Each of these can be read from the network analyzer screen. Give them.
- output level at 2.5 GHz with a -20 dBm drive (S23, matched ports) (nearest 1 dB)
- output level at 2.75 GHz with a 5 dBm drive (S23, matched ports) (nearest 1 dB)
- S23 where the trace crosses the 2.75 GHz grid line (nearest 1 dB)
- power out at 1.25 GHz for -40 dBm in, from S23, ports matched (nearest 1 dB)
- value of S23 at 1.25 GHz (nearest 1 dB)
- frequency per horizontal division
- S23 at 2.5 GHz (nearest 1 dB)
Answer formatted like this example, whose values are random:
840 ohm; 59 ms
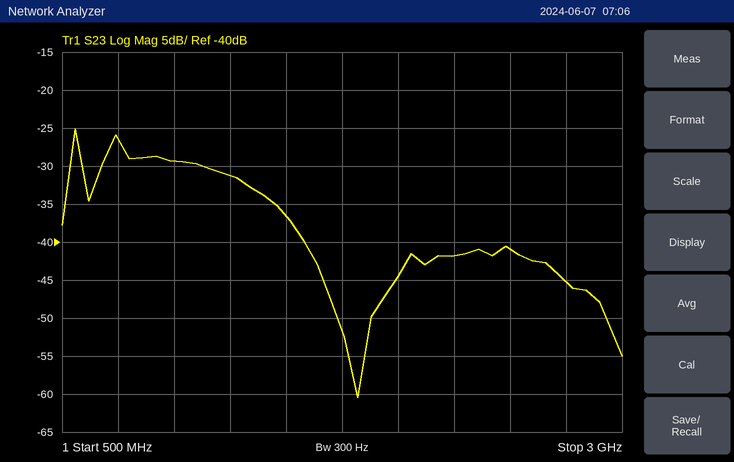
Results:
-61 dBm; -40 dBm; -45 dB; -71 dBm; -31 dB; 250 MHz; -41 dB
